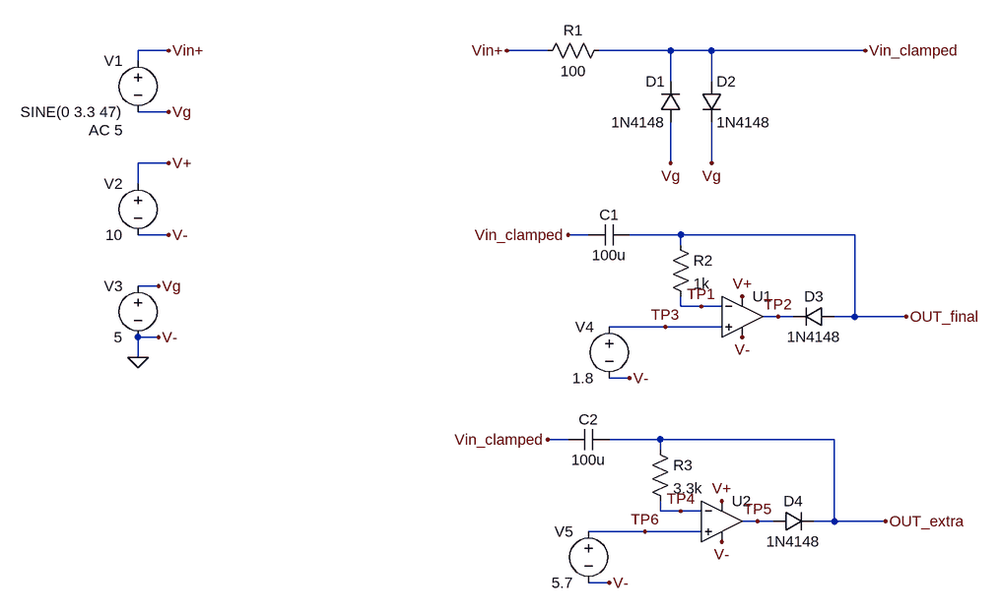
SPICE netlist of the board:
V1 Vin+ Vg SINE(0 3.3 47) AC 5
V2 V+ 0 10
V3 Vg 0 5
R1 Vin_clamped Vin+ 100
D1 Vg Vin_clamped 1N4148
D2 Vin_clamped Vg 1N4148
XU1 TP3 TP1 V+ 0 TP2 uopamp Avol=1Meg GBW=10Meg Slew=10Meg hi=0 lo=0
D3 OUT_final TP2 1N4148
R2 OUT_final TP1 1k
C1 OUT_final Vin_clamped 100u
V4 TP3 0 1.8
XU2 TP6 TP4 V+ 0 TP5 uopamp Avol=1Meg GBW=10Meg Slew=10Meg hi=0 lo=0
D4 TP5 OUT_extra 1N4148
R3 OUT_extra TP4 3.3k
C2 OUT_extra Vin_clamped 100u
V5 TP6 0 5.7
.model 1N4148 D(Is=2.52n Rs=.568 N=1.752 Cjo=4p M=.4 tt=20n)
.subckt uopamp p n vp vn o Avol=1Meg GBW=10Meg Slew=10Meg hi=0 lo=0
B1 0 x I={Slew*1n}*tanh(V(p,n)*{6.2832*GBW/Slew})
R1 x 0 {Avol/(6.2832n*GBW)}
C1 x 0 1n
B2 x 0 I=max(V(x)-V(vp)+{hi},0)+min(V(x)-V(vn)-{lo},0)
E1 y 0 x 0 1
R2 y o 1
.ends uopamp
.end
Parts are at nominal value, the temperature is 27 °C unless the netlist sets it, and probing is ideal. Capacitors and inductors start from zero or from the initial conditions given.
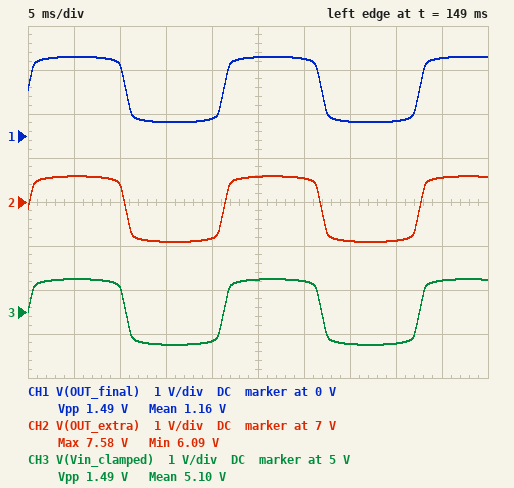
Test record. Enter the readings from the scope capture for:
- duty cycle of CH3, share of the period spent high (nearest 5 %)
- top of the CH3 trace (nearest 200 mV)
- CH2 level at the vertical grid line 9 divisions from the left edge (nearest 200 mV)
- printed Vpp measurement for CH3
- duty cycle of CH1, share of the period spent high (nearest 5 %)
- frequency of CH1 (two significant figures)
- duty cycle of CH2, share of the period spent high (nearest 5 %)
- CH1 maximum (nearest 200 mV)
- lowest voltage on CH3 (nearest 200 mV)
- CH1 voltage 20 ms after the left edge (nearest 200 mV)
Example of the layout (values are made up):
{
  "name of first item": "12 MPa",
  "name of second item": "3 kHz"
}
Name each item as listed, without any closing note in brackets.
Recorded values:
{
  "duty cycle of CH3, share of the period spent high": "50 %",
  "top of the CH3 trace": "5.8 V",
  "CH2 level at the vertical grid line 9 divisions from the left edge": "7.6 V",
  "printed Vpp measurement for CH3": "1.49 V",
  "duty cycle of CH1, share of the period spent high": "50 %",
  "frequency of CH1": "47 Hz",
  "duty cycle of CH2, share of the period spent high": "50 %",
  "CH1 maximum": "1.8 V",
  "lowest voltage on CH3": "4.2 V",
  "CH1 voltage 20 ms after the left edge": "400 mV"
}
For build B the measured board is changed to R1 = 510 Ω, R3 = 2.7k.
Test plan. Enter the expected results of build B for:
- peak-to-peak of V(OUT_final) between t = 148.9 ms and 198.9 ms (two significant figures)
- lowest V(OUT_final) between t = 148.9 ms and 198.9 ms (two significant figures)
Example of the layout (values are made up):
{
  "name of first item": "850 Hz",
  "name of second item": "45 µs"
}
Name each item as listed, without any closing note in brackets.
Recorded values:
{
  "peak-to-peak of V(OUT_final) between t = 148.9 ms and 198.9 ms": "1.3 V",
  "lowest V(OUT_final) between t = 148.9 ms and 198.9 ms": "480 mV"
}
